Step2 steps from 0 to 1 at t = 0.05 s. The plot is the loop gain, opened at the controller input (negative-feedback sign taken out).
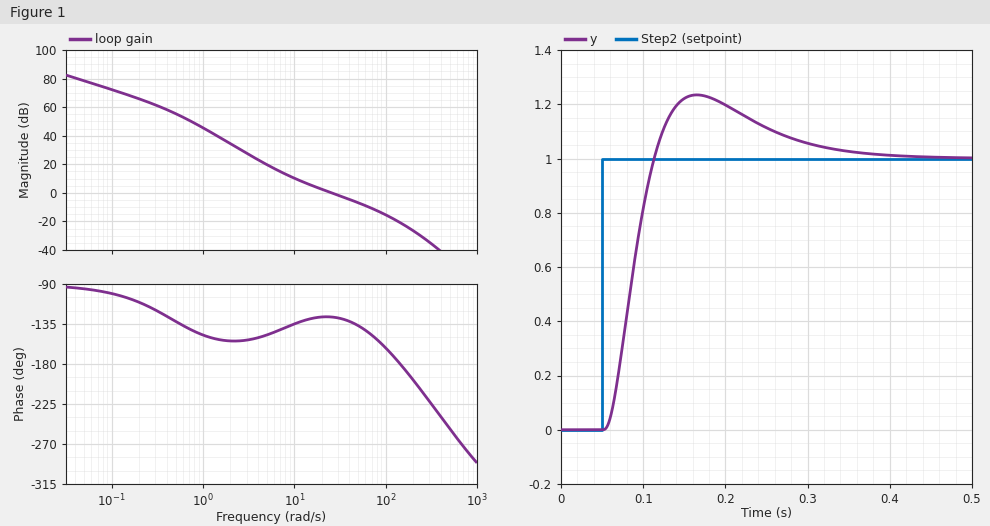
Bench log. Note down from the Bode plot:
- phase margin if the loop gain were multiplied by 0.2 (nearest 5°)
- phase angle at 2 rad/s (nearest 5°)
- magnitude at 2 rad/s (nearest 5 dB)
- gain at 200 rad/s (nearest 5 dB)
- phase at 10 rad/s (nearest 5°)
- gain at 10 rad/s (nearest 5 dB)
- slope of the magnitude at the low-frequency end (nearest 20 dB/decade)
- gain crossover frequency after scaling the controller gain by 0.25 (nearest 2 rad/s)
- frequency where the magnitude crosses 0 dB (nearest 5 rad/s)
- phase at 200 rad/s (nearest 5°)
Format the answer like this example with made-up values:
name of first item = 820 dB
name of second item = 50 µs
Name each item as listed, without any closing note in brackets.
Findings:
phase margin if the loop gain were multiplied by 0.2 = 40°
phase angle at 2 rad/s = -155°
magnitude at 2 rad/s = 35 dB
gain at 200 rad/s = -25 dB
phase at 10 rad/s = -135°
gain at 10 rad/s = 10 dB
slope of the magnitude at the low-frequency end = -20 dB/decade
gain crossover frequency after scaling the controller gain by 0.25 = 8 rad/s
frequency where the magnitude crosses 0 dB = 25 rad/s
phase at 200 rad/s = -200°
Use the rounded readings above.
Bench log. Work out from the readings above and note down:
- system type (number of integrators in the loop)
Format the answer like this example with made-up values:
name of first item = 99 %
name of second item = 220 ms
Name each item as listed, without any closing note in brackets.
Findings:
system type = 1
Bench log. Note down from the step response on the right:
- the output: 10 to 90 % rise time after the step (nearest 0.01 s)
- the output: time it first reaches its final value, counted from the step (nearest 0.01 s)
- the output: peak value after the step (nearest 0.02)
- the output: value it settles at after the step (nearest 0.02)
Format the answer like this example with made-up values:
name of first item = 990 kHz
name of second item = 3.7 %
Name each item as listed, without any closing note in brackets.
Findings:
the output: 10 to 90 % rise time after the step = 0.04 s
the output: time it first reaches its final value, counted from the step = 0.06 s
the output: peak value after the step = 1.24
the output: value it settles at after the step = 1.00
